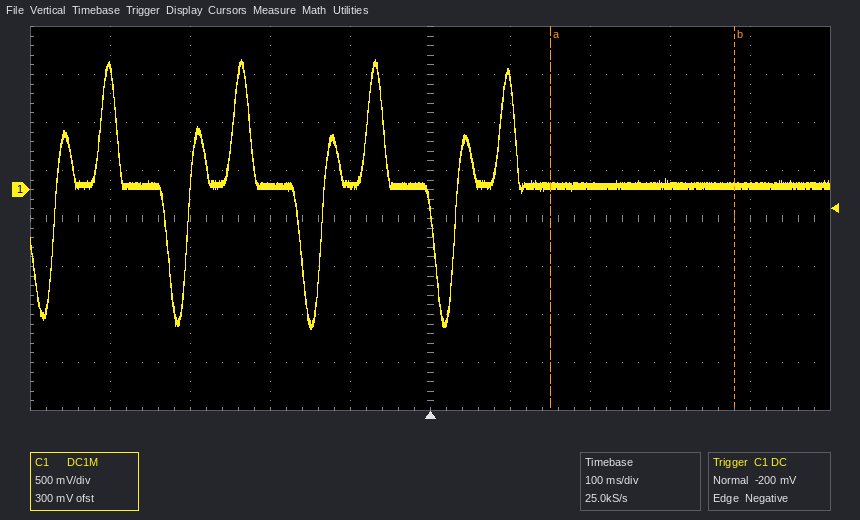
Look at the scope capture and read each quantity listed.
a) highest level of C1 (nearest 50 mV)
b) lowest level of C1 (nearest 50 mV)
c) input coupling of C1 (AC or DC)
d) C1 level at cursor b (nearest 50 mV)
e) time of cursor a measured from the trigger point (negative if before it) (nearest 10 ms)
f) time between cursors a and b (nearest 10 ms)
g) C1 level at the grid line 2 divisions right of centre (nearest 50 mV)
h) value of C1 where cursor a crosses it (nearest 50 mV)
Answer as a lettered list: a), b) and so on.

a) 1.35 V
b) -1.45 V
c) DC
d) 50 mV
e) +150 ms
f) 230 ms
g) 50 mV
h) 50 mV
